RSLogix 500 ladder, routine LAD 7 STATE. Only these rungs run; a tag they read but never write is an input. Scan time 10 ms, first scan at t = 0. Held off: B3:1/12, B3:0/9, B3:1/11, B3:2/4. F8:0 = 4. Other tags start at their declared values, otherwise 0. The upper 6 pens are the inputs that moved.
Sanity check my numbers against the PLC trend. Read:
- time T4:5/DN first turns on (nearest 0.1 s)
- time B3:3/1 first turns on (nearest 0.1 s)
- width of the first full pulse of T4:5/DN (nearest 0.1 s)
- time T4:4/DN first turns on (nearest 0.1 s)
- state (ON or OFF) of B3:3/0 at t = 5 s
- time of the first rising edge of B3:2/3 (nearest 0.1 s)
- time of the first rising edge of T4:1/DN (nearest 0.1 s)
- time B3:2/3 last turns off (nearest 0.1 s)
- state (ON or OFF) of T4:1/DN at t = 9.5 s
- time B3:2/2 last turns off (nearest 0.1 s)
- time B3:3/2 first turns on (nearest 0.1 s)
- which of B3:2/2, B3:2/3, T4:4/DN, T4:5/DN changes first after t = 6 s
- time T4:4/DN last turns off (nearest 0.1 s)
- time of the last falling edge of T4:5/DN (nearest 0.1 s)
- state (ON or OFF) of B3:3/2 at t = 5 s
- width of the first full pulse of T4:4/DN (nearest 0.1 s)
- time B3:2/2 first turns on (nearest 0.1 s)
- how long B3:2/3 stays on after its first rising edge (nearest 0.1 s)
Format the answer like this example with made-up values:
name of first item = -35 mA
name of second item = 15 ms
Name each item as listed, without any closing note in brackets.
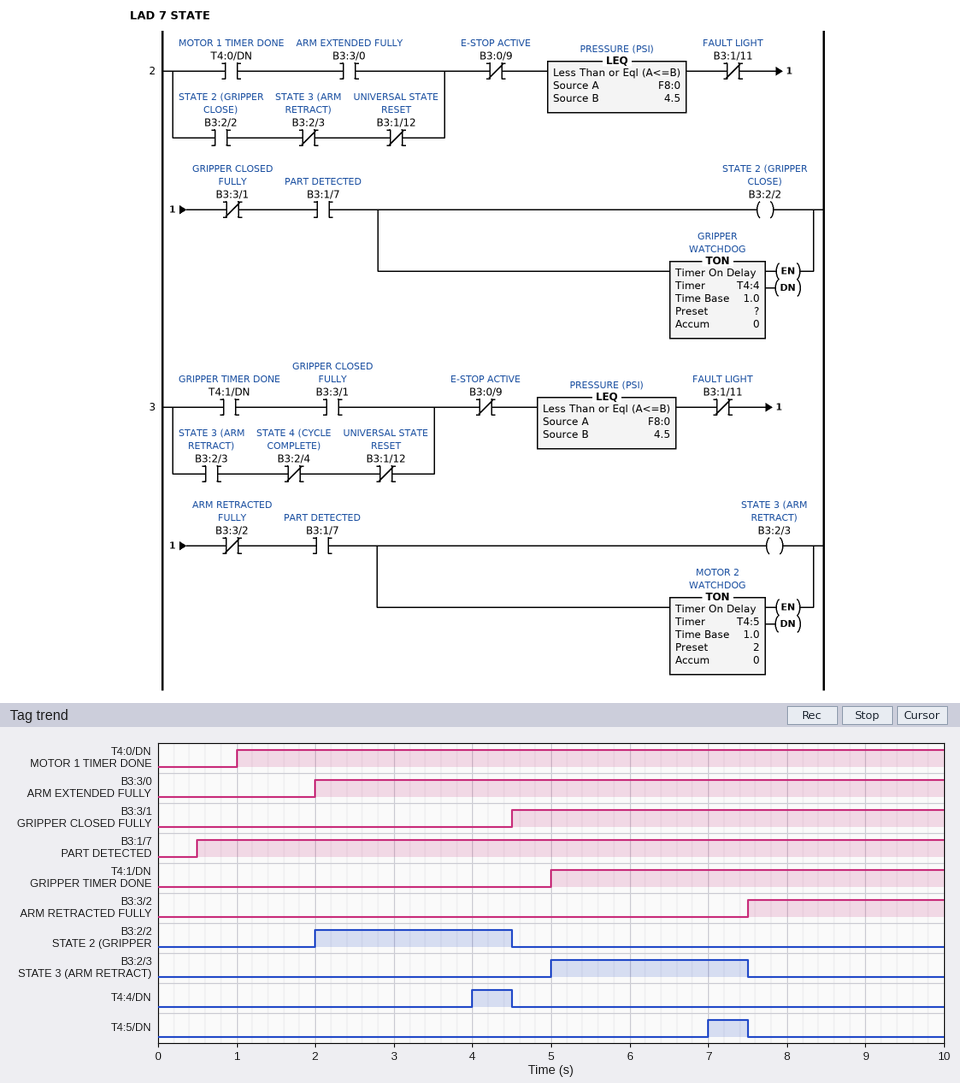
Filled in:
time T4:5/DN first turns on = 7.0 s
time B3:3/1 first turns on = 4.5 s
width of the first full pulse of T4:5/DN = 0.5 s
time T4:4/DN first turns on = 4.0 s
state (ON or OFF) of B3:3/0 at t = 5 s = ON
time of the first rising edge of B3:2/3 = 5.0 s
time of the first rising edge of T4:1/DN = 5.0 s
time B3:2/3 last turns off = 7.5 s
state (ON or OFF) of T4:1/DN at t = 9.5 s = ON
time B3:2/2 last turns off = 4.5 s
time B3:3/2 first turns on = 7.5 s
which of B3:2/2, B3:2/3, T4:4/DN, T4:5/DN changes first after t = 6 s = T4:5/DN
time T4:4/DN last turns off = 4.5 s
time of the last falling edge of T4:5/DN = 7.5 s
state (ON or OFF) of B3:3/2 at t = 5 s = OFF
width of the first full pulse of T4:4/DN = 0.5 s
time B3:2/2 first turns on = 2.0 s
how long B3:2/3 stays on after its first rising edge = 2.5 s
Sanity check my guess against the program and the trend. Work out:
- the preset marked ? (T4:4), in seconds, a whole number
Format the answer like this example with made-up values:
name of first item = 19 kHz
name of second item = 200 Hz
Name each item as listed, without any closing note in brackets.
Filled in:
the preset marked ? (T4:4), in seconds, a whole number = 2 s
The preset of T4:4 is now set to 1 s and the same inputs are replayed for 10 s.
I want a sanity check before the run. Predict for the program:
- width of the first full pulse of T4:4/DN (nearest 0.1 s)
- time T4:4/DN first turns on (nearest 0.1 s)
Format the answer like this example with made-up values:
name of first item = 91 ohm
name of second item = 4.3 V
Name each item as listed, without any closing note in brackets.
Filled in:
width of the first full pulse of T4:4/DN = 1.5 s
time T4:4/DN first turns on = 3.0 s
